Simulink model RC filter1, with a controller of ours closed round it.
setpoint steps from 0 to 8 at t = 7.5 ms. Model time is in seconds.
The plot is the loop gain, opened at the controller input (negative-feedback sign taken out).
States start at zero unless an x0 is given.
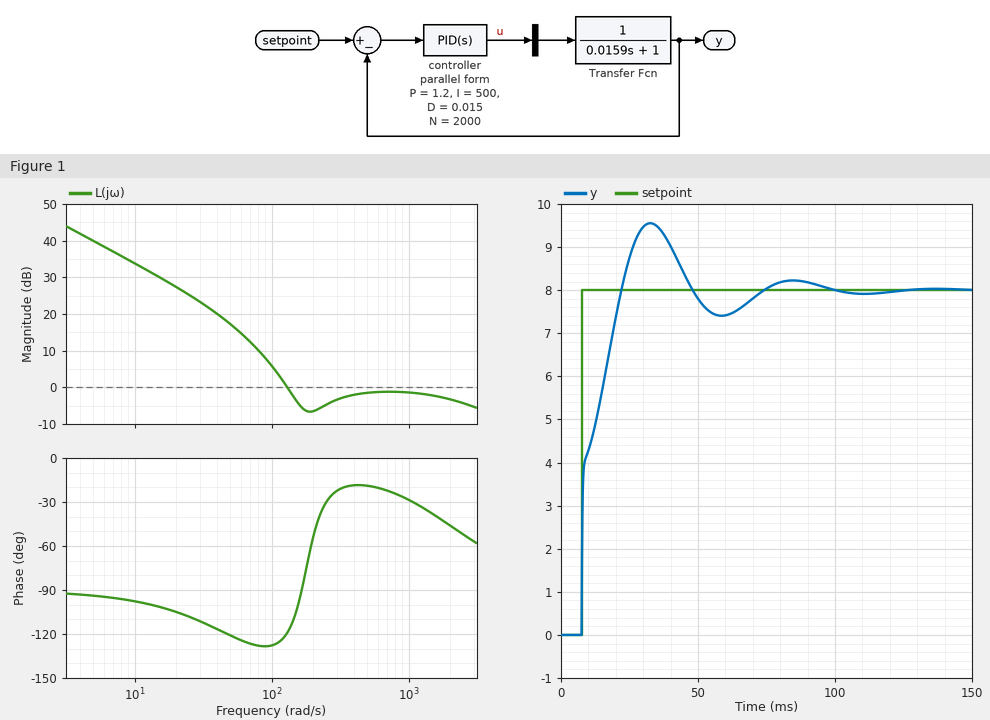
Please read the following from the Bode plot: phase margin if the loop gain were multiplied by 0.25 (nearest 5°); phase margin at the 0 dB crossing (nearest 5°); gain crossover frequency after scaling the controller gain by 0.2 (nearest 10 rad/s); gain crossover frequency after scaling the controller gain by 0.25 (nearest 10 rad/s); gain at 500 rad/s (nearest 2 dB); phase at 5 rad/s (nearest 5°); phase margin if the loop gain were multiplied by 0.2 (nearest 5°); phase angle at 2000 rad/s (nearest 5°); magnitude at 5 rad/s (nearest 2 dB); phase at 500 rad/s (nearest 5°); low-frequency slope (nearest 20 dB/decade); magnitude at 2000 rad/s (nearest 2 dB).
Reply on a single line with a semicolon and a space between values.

55°; 60°; 60 rad/s; 70 rad/s; -2 dB; -95°; 55°; -45°; 40 dB; -20°; -20 dB/decade; -4 dB
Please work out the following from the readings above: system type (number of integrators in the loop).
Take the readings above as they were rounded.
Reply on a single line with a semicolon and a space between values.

1
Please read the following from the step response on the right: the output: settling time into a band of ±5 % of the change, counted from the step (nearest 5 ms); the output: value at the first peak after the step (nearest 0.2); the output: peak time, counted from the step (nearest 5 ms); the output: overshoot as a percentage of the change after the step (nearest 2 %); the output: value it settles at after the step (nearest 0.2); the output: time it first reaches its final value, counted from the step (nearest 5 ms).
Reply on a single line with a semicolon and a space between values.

60 ms; 9.6; 25 ms; 20 %; 8.0; 15 ms
